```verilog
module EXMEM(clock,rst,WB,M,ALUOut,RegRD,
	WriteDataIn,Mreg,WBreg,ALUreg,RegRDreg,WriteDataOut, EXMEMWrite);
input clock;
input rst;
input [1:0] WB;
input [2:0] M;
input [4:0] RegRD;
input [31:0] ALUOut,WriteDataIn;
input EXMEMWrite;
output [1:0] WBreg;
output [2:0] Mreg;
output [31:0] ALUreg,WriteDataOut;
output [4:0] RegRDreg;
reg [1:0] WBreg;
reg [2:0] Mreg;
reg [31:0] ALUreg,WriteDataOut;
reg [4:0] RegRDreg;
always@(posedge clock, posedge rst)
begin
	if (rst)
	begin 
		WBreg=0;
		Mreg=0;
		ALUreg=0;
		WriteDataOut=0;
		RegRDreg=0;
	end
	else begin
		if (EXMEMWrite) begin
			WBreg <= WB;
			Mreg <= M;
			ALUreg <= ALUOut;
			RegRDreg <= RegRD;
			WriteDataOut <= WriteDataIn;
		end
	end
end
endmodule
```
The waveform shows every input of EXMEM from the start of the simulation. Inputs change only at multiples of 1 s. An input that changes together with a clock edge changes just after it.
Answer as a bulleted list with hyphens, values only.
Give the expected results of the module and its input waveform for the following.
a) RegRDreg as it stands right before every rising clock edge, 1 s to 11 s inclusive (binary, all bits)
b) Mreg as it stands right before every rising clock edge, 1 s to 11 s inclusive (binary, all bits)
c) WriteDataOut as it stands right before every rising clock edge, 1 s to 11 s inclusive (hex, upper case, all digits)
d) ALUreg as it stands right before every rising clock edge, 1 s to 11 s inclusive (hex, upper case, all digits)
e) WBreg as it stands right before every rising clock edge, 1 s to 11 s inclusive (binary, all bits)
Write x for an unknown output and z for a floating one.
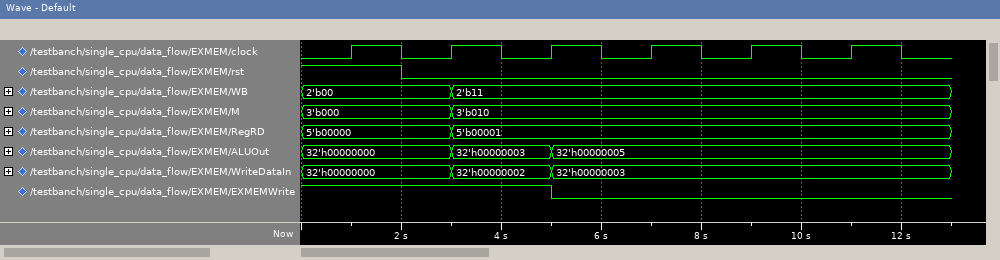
- 00000, 00000, 00000, 00001, 00001, 00001
- 000, 000, 000, 010, 010, 010
- 00000000, 00000000, 00000000, 00000002, 00000002, 00000002
- 00000000, 00000000, 00000000, 00000003, 00000003, 00000003
- 00, 00, 00, 11, 11, 11
